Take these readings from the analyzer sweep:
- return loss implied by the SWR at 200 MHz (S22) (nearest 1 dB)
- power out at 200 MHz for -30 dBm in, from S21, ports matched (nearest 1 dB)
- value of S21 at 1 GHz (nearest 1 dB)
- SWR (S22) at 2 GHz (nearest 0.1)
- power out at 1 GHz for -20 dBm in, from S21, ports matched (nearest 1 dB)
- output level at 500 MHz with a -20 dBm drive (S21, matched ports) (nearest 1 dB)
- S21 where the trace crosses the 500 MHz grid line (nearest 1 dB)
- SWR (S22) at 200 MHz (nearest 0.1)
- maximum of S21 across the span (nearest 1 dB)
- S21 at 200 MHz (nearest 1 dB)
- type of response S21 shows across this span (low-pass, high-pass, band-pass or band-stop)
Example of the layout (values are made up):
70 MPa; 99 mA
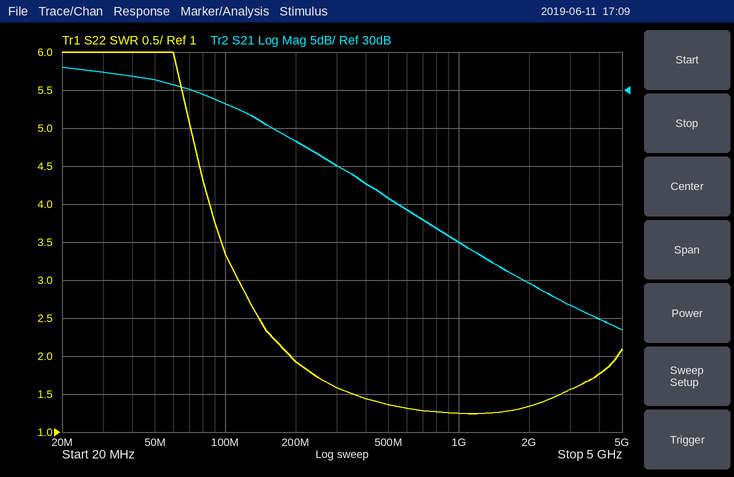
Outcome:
10 dB; -7 dBm; 10 dB; 1.3; -10 dBm; -4 dBm; 16 dB; 1.9; 33 dB; 23 dB; low-pass
